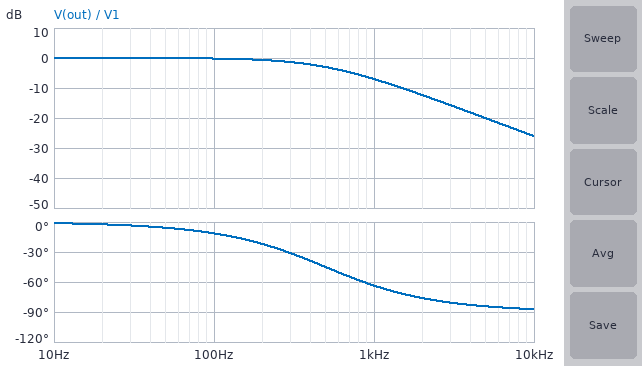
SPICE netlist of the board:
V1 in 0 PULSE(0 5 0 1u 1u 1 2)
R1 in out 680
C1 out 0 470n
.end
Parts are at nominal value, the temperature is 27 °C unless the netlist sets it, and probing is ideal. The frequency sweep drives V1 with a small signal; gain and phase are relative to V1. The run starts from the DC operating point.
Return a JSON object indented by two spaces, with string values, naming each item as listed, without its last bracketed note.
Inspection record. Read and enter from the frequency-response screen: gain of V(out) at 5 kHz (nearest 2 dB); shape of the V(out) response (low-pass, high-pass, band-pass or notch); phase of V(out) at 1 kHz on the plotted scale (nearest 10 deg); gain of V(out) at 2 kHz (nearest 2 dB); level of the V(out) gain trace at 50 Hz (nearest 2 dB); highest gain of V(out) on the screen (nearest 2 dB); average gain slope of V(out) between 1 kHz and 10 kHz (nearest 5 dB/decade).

{
  "gain of V(out) at 5 kHz": "-20 dB",
  "shape of the V(out) response": "low-pass",
  "phase of V(out) at 1 kHz on the plotted scale": "-60 deg",
  "gain of V(out) at 2 kHz": "-12 dB",
  "level of the V(out) gain trace at 50 Hz": "0 dB",
  "highest gain of V(out) on the screen": "0 dB",
  "average gain slope of V(out) between 1 kHz and 10 kHz": "-20 dB/decade"
}
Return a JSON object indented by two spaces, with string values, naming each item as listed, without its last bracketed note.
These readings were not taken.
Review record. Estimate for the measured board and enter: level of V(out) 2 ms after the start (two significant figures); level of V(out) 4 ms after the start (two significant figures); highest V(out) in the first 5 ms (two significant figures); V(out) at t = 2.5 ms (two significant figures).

{
  "level of V(out) 2 ms after the start": "5.0 V",
  "level of V(out) 4 ms after the start": "5.0 V",
  "highest V(out) in the first 5 ms": "5.0 V",
  "V(out) at t = 2.5 ms": "5.0 V"
}
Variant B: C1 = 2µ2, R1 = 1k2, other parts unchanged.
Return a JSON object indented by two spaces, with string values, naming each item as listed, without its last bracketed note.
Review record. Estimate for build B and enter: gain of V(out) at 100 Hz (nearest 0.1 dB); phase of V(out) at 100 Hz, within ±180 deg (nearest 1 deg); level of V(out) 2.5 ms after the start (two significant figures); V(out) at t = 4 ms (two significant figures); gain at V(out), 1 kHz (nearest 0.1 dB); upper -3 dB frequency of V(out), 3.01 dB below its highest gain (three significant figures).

{
  "gain of V(out) at 100 Hz": "-5.7 dB",
  "phase of V(out) at 100 Hz, within ±180 deg": "-59 deg",
  "level of V(out) 2.5 ms after the start": "3.1 V",
  "V(out) at t = 4 ms": "3.9 V",
  "gain at V(out), 1 kHz": "-24.4 dB",
  "upper -3 dB frequency of V(out), 3.01 dB below its highest gain": "60.3 Hz"
}
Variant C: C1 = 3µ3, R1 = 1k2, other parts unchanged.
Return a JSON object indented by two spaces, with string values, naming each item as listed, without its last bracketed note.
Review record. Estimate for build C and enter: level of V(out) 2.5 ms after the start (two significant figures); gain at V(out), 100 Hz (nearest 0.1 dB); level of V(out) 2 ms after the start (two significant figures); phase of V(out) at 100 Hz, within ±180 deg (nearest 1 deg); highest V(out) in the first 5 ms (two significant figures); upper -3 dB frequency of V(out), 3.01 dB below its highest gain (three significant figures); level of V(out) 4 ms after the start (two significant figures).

{
  "level of V(out) 2.5 ms after the start": "2.3 V",
  "gain at V(out), 100 Hz": "-8.6 dB",
  "level of V(out) 2 ms after the start": "2.0 V",
  "phase of V(out) at 100 Hz, within ±180 deg": "-68 deg",
  "highest V(out) in the first 5 ms": "3.6 V",
  "upper -3 dB frequency of V(out), 3.01 dB below its highest gain": "40.2 Hz",
  "level of V(out) 4 ms after the start": "3.2 V"
}
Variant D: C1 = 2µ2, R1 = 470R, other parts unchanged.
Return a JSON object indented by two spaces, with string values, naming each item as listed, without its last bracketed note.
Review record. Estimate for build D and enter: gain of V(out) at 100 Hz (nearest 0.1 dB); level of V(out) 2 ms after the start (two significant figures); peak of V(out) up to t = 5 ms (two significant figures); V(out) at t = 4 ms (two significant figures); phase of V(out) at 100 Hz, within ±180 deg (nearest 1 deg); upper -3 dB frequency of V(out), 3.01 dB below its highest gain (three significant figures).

{
  "gain of V(out) at 100 Hz": "-1.5 dB",
  "level of V(out) 2 ms after the start": "4.3 V",
  "peak of V(out) up to t = 5 ms": "5.0 V",
  "V(out) at t = 4 ms": "4.9 V",
  "phase of V(out) at 100 Hz, within ±180 deg": "-33 deg",
  "upper -3 dB frequency of V(out), 3.01 dB below its highest gain": "154 Hz"
}
